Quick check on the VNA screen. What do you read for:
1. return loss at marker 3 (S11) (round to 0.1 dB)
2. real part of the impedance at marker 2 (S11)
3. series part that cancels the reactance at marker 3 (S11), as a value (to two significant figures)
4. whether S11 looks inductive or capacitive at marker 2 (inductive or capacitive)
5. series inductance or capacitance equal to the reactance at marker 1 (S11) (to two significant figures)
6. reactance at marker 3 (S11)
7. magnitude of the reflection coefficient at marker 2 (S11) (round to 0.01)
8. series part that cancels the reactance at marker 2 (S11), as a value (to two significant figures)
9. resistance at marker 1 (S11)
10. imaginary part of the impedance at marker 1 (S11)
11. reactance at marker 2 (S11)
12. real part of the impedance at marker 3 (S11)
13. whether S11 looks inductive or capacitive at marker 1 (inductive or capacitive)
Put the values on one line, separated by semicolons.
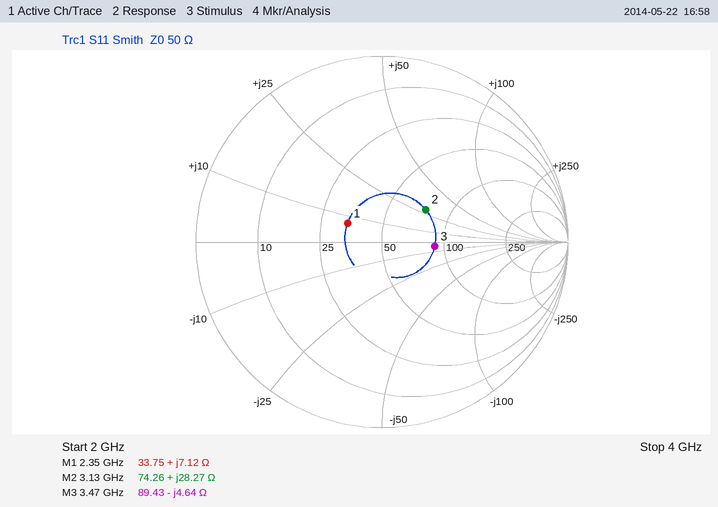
10.9 dB; 74.26 Ω; 210 pH; inductive; 480 pH; -4.64 Ω; 0.29; 1.8 pF; 33.75 Ω; +7.12 Ω; +28.27 Ω; 89.43 Ω; inductive
